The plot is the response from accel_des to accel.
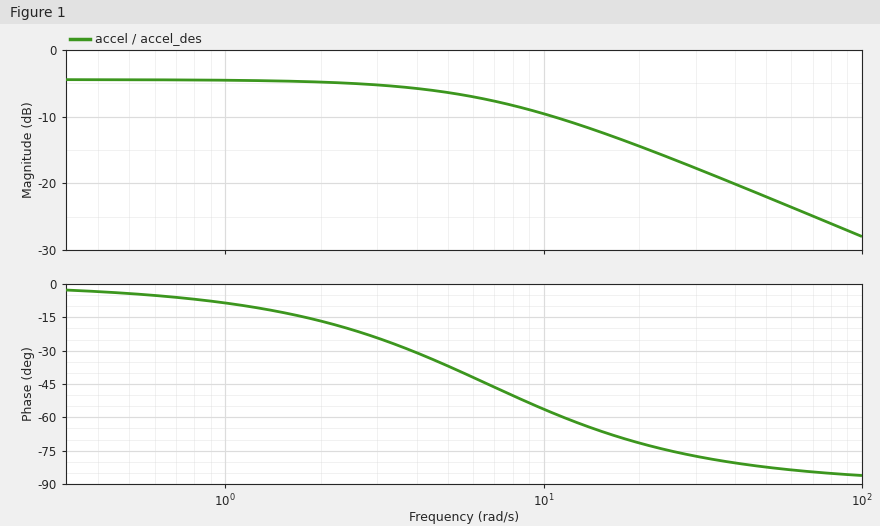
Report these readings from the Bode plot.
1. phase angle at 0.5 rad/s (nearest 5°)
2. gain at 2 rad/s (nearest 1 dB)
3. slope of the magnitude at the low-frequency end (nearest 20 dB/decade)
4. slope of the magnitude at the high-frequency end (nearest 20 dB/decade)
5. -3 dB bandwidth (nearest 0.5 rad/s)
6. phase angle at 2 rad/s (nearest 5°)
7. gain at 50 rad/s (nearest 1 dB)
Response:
-5°
-5 dB
0 dB/decade
-20 dB/decade
6.5 rad/s
-15°
-22 dB
